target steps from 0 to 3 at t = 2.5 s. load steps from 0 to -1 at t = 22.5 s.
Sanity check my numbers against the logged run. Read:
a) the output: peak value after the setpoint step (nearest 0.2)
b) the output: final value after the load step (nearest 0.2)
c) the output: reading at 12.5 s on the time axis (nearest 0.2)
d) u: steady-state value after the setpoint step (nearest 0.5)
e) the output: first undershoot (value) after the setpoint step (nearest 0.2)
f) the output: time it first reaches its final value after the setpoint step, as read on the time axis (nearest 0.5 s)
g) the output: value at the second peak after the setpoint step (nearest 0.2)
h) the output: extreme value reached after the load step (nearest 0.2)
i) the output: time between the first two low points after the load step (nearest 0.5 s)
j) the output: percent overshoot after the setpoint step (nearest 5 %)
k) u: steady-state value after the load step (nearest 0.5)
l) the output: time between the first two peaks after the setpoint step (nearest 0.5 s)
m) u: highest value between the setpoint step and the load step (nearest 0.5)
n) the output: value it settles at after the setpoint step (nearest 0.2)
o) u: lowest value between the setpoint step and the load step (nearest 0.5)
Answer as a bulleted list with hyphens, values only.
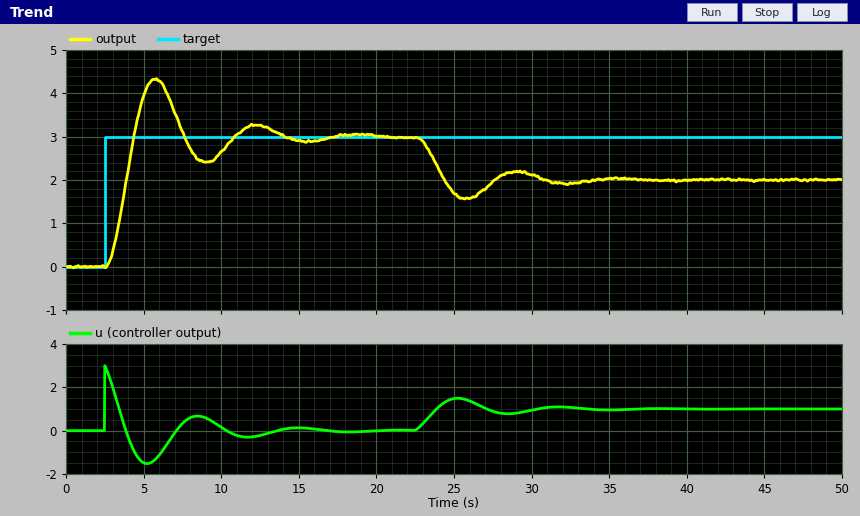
- 4.4
- 2.0
- 3.2
- 0.0
- 2.4
- 4.5 s
- 3.2
- 1.6
- 6.5 s
- 45 %
- 1.0
- 6.5 s
- 3.0
- 3.0
- -1.5
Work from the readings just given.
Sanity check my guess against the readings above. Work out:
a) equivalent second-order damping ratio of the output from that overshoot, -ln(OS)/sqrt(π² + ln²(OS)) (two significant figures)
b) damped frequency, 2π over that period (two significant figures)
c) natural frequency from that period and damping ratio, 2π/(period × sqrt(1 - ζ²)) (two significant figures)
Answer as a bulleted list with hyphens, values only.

- 0.25
- 0.97 rad/s
- 1.00 rad/s
